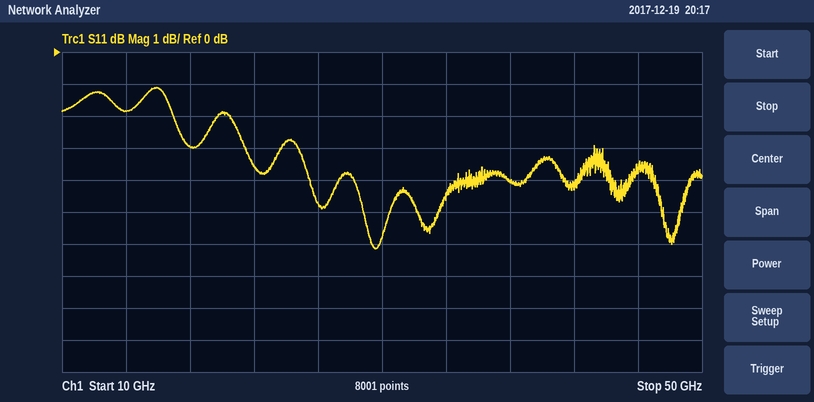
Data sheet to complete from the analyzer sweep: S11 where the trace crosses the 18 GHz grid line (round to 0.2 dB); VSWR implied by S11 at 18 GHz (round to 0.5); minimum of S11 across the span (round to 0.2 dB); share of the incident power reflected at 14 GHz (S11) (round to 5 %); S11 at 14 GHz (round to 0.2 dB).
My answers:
-3.0 dB
6.0
-6.2 dB
65 %
-1.8 dB
